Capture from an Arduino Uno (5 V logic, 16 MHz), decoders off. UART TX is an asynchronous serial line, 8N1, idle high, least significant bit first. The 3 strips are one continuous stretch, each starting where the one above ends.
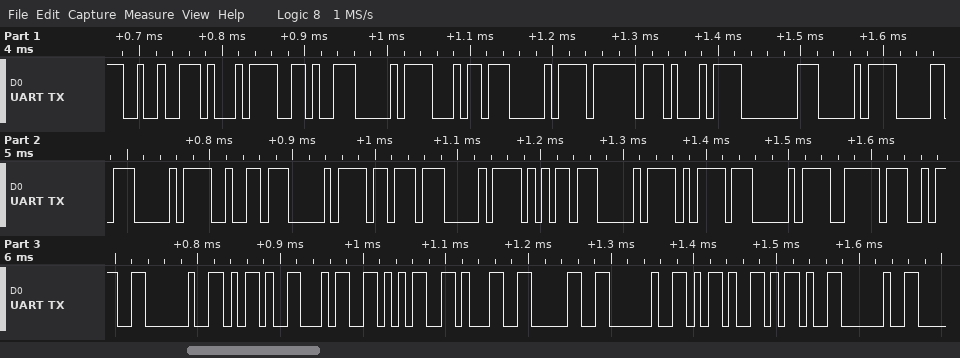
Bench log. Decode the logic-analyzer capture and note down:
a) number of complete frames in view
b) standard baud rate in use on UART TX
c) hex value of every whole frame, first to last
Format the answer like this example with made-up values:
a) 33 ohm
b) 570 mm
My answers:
a) 32
b) 115200 baud
c) 92 D1 96 D0 B4 D0 BF D1 80 D0 B0 D0 B2 D0 BB D0 B5 D0 BD D0 BE 3A 20 2D 34 35 31 30 20 2D 2D 20
